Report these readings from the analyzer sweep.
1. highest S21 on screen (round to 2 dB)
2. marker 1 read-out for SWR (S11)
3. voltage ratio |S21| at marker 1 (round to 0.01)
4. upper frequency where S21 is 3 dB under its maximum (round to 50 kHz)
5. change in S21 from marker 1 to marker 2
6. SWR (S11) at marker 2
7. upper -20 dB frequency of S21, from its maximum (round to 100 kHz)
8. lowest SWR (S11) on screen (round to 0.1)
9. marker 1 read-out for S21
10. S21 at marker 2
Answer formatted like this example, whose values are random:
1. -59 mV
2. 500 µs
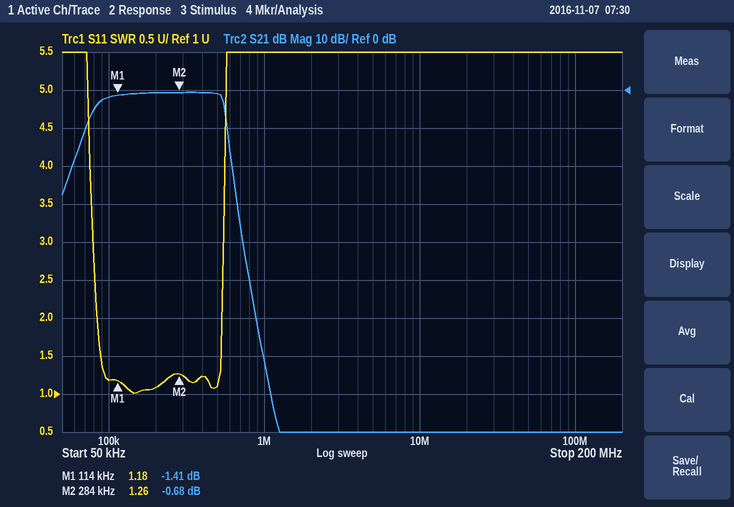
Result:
1. 0 dB
2. 1.18
3. 0.85
4. 550 kHz
5. 0.73 dB
6. 1.26
7. 600 kHz
8. 1.0
9. -1.41 dB
10. -0.68 dB
